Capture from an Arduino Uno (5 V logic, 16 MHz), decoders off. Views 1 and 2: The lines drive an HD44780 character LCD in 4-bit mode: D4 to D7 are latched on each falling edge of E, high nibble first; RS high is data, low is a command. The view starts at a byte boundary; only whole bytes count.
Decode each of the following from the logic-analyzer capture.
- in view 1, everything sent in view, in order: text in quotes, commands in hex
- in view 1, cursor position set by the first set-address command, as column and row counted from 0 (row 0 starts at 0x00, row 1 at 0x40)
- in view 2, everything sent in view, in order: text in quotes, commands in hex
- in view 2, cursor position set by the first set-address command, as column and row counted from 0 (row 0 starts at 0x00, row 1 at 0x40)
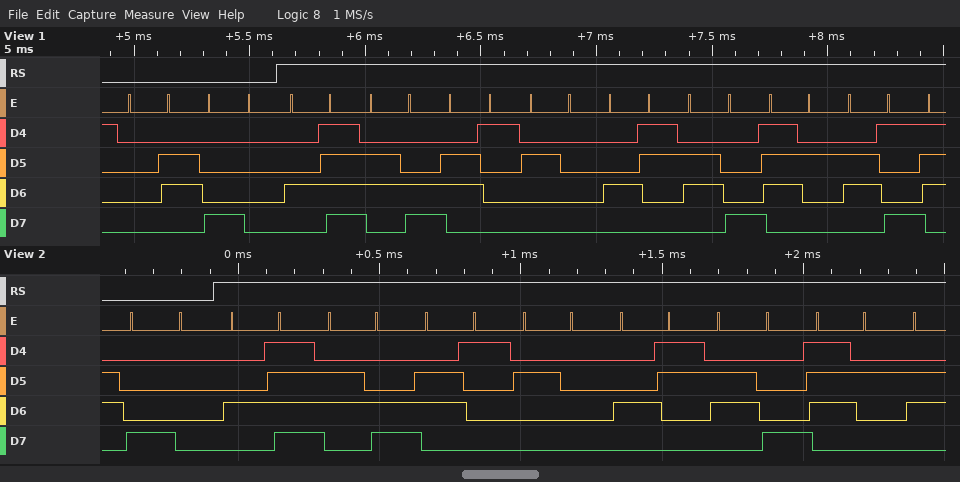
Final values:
0x06 0x80 "Ola Chri"
column 0, row 0
0x80 "Ola Chr"
column 0, row 0
